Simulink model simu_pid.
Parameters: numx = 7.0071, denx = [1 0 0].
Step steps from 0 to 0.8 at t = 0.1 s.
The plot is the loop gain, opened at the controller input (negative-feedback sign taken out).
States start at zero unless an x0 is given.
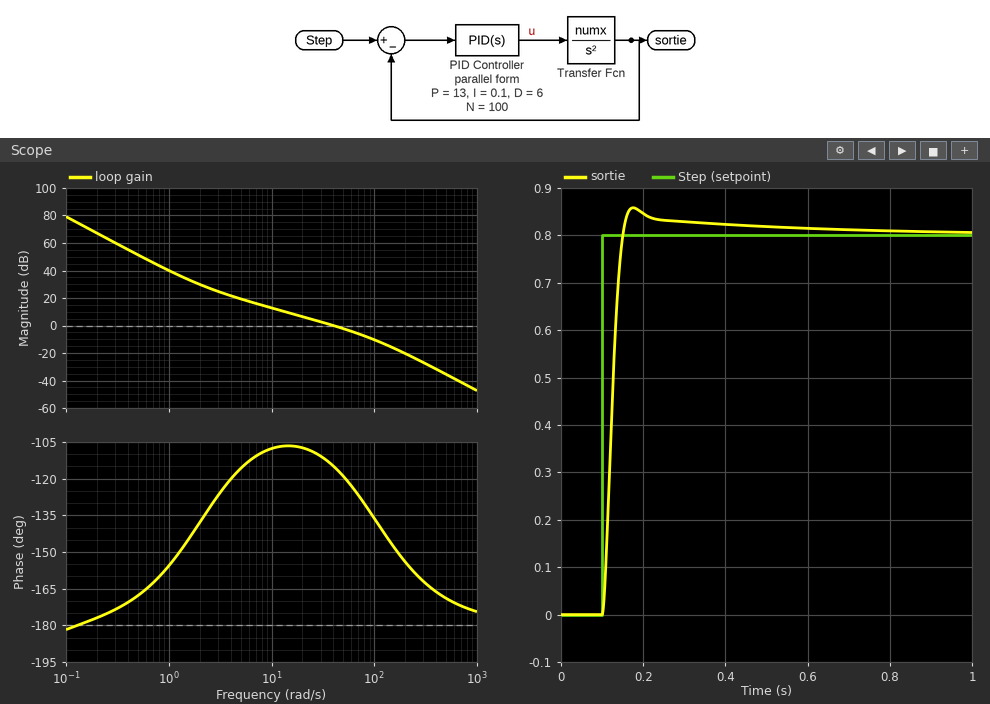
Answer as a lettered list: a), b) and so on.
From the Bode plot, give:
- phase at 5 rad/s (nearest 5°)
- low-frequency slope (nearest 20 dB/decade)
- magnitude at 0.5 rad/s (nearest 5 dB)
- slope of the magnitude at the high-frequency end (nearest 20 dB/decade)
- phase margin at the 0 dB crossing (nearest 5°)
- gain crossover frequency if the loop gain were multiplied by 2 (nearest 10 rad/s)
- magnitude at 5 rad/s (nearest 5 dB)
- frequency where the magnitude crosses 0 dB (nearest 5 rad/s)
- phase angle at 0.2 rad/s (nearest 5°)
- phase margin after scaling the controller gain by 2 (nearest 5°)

a) -115°
b) -40 dB/decade
c) 50 dB
d) -40 dB/decade
e) 65°
f) 70 rad/s
g) 20 dB
h) 40 rad/s
i) -175°
j) 55°
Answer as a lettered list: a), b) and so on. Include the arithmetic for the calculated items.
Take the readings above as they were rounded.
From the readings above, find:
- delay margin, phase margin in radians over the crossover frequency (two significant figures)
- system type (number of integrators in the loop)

a) 65 × π / 180 / 40 = 0.028 s
b) 2
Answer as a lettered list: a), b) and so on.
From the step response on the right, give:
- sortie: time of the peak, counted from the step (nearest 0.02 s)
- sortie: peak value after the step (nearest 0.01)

a) 0.08 s
b) 0.86
